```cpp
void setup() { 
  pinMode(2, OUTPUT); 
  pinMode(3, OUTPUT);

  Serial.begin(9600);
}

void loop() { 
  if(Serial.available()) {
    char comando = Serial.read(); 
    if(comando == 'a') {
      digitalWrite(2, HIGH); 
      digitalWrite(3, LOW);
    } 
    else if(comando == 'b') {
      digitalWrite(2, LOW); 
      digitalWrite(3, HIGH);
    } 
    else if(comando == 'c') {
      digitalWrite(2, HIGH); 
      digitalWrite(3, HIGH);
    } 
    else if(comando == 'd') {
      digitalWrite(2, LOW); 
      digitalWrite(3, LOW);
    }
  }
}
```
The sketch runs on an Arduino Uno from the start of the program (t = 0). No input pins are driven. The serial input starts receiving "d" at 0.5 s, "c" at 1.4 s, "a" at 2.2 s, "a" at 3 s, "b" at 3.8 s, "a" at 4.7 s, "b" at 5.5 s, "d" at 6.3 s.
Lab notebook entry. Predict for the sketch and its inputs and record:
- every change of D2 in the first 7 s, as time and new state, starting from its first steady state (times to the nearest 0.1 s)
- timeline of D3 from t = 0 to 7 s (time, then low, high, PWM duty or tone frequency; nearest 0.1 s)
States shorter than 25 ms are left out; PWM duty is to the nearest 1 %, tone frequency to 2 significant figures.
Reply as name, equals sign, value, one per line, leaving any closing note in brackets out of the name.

every change of D2 in the first 7 s, as time and new state, starting from its first steady state = 0 s low; 1.4 s high; 3.8 s low; 4.7 s high; 5.5 s low
timeline of D3 from t = 0 to 7 s = 0 s low; 1.4 s high; 2.2 s low; 3.8 s high; 4.7 s low; 5.5 s high; 6.3 s low
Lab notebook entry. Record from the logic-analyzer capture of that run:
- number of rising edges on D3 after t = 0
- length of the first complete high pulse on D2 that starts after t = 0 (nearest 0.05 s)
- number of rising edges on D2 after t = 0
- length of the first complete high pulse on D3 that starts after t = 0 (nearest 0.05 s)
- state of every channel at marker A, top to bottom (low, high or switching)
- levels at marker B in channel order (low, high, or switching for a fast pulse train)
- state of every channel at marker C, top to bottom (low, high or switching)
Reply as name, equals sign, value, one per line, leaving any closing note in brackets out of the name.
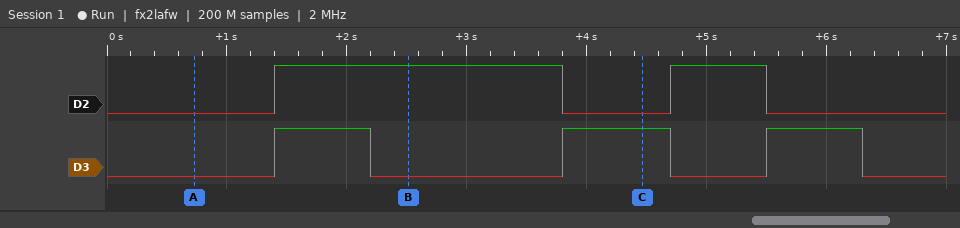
number of rising edges on D3 after t = 0 = 3
length of the first complete high pulse on D2 that starts after t = 0 = 2.40 s
number of rising edges on D2 after t = 0 = 2
length of the first complete high pulse on D3 that starts after t = 0 = 0.80 s
state of every channel at marker A, top to bottom = D2 low, D3 low
levels at marker B in channel order = D2 high, D3 low
state of every channel at marker C, top to bottom = D2 low, D3 high
